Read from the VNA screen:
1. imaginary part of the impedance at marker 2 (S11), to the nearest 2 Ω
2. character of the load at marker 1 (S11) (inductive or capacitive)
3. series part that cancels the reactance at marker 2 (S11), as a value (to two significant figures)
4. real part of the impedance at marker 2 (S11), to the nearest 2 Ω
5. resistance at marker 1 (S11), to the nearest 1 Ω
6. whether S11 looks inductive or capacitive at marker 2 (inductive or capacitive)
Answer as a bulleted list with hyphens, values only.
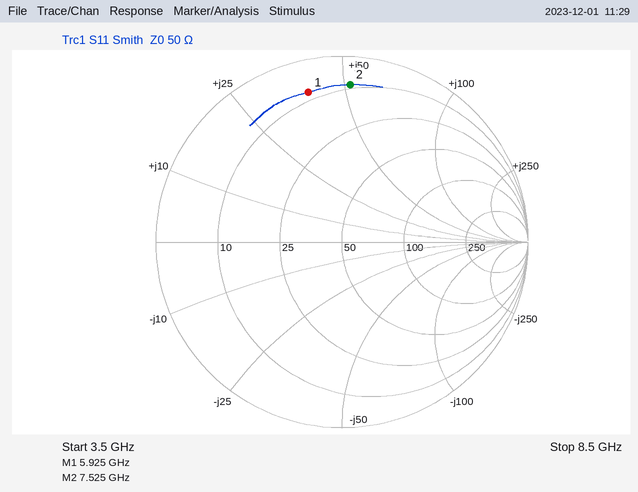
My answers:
- +52 Ω
- inductive
- 410 fF
- 8 Ω
- 8 Ω
- inductive
